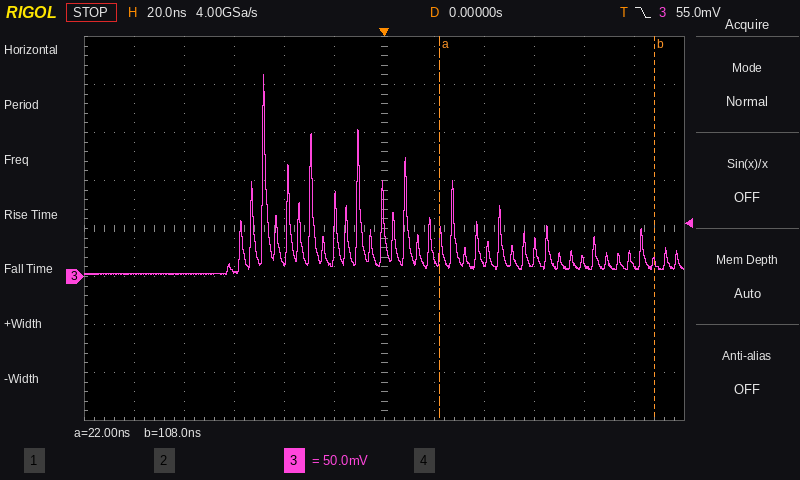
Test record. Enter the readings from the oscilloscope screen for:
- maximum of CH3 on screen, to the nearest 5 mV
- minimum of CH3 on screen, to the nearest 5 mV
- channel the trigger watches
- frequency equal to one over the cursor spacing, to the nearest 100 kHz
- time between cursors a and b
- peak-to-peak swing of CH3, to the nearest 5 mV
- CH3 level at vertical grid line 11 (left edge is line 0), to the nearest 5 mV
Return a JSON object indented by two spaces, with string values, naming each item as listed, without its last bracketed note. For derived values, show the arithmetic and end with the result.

{
  "maximum of CH3 on screen, to the nearest 5 mV": "210 mV",
  "minimum of CH3 on screen, to the nearest 5 mV": "0 mV",
  "channel the trigger watches": "CH3",
  "frequency equal to one over the cursor spacing, to the nearest 100 kHz": "1 / 86 ns ≈ 11.6 MHz",
  "time between cursors a and b": "108 ns − (22 ns) = 86 ns",
  "peak-to-peak swing of CH3, to the nearest 5 mV": "210 mV − (0 mV) = 210 mV",
  "CH3 level at vertical grid line 11 (left edge is line 0), to the nearest 5 mV": "10 mV"
}
